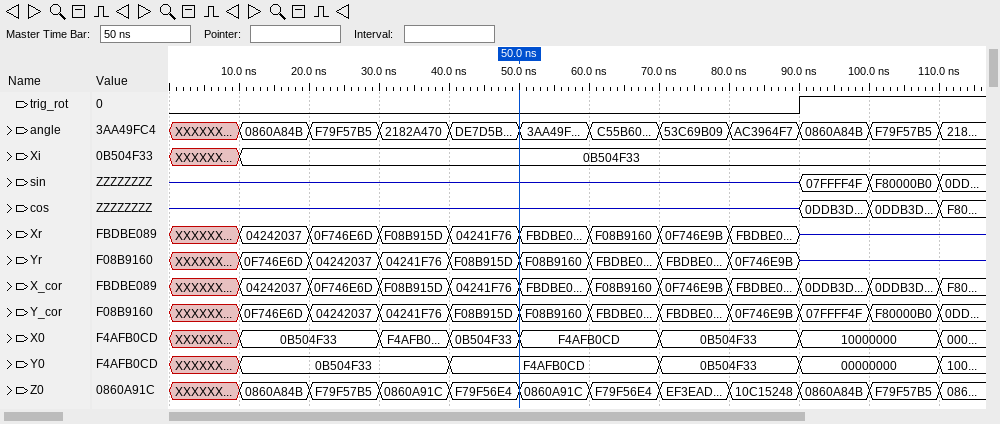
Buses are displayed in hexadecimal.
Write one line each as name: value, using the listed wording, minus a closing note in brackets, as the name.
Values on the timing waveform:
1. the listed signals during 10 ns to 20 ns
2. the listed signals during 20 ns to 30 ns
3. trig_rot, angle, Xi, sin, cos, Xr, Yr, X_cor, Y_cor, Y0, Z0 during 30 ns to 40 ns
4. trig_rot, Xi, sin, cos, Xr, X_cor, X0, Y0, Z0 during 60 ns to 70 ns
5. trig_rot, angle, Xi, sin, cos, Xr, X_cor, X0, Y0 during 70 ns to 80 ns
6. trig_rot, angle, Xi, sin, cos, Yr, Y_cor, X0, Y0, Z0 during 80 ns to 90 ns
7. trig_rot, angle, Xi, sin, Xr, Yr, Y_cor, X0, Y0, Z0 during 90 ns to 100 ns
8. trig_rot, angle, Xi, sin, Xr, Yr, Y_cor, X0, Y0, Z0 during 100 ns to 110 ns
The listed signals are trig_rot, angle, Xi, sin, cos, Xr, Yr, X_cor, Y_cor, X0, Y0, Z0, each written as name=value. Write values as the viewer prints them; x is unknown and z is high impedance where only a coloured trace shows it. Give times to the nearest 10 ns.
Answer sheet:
the listed signals during 10 ns to 20 ns: trig_rot=0, angle=0860A84B, Xi=0B504F33, sin=z, cos=z, Xr=04242037, Yr=0F746E6D, X_cor=04242037, Y_cor=0F746E6D, X0=0B504F33, Y0=0B504F33, Z0=0860A84B
the listed signals during 20 ns to 30 ns: trig_rot=0, angle=F79F57B5, Xi=0B504F33, sin=z, cos=z, Xr=0F746E6D, Yr=04242037, X_cor=0F746E6D, Y_cor=04242037, X0=0B504F33, Y0=0B504F33, Z0=F79F57B5
trig_rot, angle, Xi, sin, cos, Xr, Yr, X_cor, Y_cor, Y0, Z0 during 30 ns to 40 ns: trig_rot=0, angle=2182A470, Xi=0B504F33, sin=z, cos=z, Xr=F08B915D, Yr=04241F76, X_cor=F08B915D, Y_cor=04241F76, Y0=0B504F33, Z0=0860A91C
trig_rot, Xi, sin, cos, Xr, X_cor, X0, Y0, Z0 during 60 ns to 70 ns: trig_rot=0, Xi=0B504F33, sin=z, cos=z, Xr=F08B9160, X_cor=F08B9160, X0=F4AFB0CD, Y0=F4AFB0CD, Z0=F79F56E4
trig_rot, angle, Xi, sin, cos, Xr, X_cor, X0, Y0 during 70 ns to 80 ns: trig_rot=0, angle=53C69B09, Xi=0B504F33, sin=z, cos=z, Xr=0F746E9B, X_cor=0F746E9B, X0=0B504F33, Y0=0B504F33
trig_rot, angle, Xi, sin, cos, Yr, Y_cor, X0, Y0, Z0 during 80 ns to 90 ns: trig_rot=0, angle=AC3964F7, Xi=0B504F33, sin=z, cos=z, Yr=0F746E9B, Y_cor=0F746E9B, X0=0B504F33, Y0=0B504F33, Z0=10C15248
trig_rot, angle, Xi, sin, Xr, Yr, Y_cor, X0, Y0, Z0 during 90 ns to 100 ns: trig_rot=1, angle=0860A84B, Xi=0B504F33, sin=07FFFF4F, Xr=z, Yr=z, Y_cor=07FFFF4F, X0=10000000, Y0=00000000, Z0=0860A84B
trig_rot, angle, Xi, sin, Xr, Yr, Y_cor, X0, Y0, Z0 during 100 ns to 110 ns: trig_rot=1, angle=F79F57B5, Xi=0B504F33, sin=F80000B0, Xr=z, Yr=z, Y_cor=F80000B0, X0=10000000, Y0=00000000, Z0=F79F57B5
